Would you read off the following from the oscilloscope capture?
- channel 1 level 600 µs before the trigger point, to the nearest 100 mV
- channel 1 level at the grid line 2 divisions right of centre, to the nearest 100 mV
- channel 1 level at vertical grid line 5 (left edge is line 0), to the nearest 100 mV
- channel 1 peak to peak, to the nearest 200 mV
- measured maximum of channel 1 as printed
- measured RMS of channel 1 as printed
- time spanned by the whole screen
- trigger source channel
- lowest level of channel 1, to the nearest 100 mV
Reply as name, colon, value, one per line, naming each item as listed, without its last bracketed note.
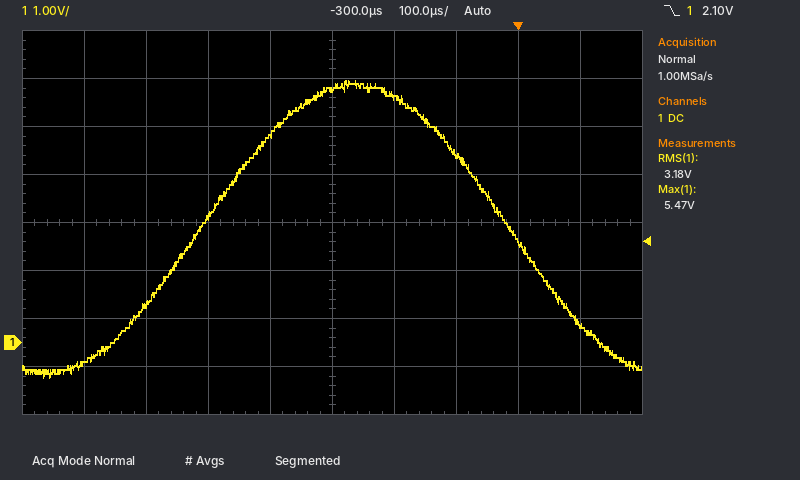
channel 1 level 600 µs before the trigger point, to the nearest 100 mV: 800 mV
channel 1 level at the grid line 2 divisions right of centre, to the nearest 100 mV: 3.9 V
channel 1 level at vertical grid line 5 (left edge is line 0), to the nearest 100 mV: 5.3 V
channel 1 peak to peak, to the nearest 200 mV: 6.2 V
measured maximum of channel 1 as printed: 5.47 V
measured RMS of channel 1 as printed: 3.18 V
time spanned by the whole screen: 1 ms
trigger source channel: channel 1
lowest level of channel 1, to the nearest 100 mV: -700 mV
